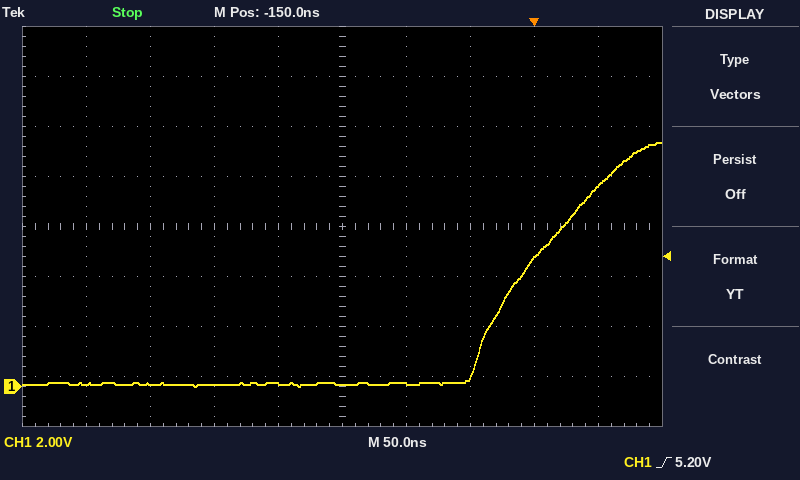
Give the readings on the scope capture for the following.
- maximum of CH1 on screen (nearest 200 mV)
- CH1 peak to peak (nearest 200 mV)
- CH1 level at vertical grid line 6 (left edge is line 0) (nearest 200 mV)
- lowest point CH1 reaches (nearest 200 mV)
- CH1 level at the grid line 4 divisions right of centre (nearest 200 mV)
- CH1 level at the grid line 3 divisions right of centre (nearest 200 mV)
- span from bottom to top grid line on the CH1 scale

9.8 V
9.8 V
200 mV
0.0 V
8.0 V
5.2 V
16 V
